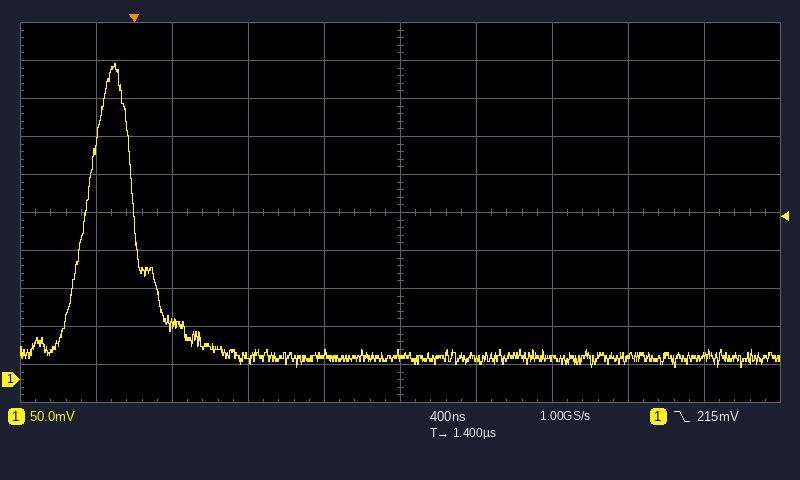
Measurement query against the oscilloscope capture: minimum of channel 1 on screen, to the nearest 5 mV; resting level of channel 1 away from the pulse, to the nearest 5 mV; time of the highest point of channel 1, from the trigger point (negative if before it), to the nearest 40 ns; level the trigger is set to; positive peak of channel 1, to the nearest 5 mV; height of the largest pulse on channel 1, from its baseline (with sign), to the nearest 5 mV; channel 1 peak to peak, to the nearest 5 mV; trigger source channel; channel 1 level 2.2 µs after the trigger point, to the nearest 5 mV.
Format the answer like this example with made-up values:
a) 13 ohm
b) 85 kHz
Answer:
a) 15 mV
b) 30 mV
c) -120 ns
d) 215 mV
e) 415 mV
f) +385 mV
g) 400 mV
h) channel 1
i) 30 mV
